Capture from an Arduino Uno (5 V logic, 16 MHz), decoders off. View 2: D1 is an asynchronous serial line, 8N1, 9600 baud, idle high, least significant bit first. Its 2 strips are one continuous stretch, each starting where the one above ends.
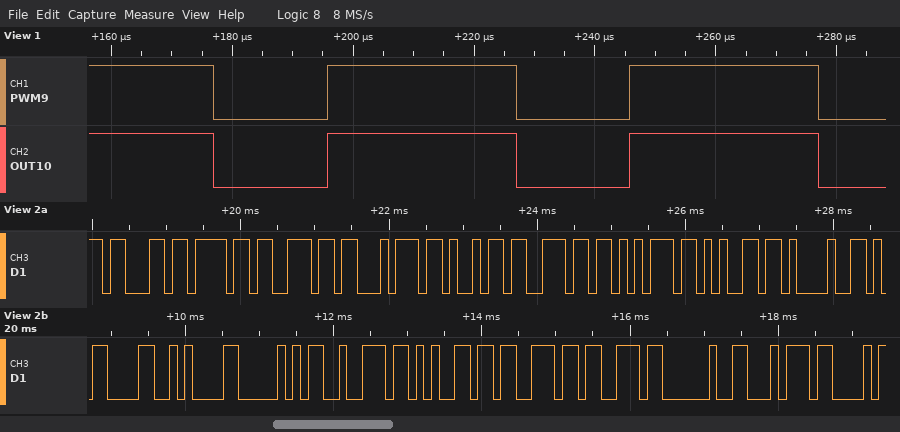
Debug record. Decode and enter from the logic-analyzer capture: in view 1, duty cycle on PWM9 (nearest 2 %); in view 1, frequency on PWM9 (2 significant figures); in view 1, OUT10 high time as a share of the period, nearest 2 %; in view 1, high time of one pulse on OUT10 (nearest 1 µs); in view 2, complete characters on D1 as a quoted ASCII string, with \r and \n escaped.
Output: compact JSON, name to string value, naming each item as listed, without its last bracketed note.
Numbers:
{"in view 1, duty cycle on PWM9": "62 %", "in view 1, frequency on PWM9": "20 kHz", "in view 1, OUT10 high time as a share of the period, nearest 2 %": "62 %", "in view 1, high time of one pulse on OUT10": "31 µs", "in view 2, complete characters on D1 as a quoted ASCII string, with \\r and \\n escaped": "\"continue!\\r\\nPress t\""}
